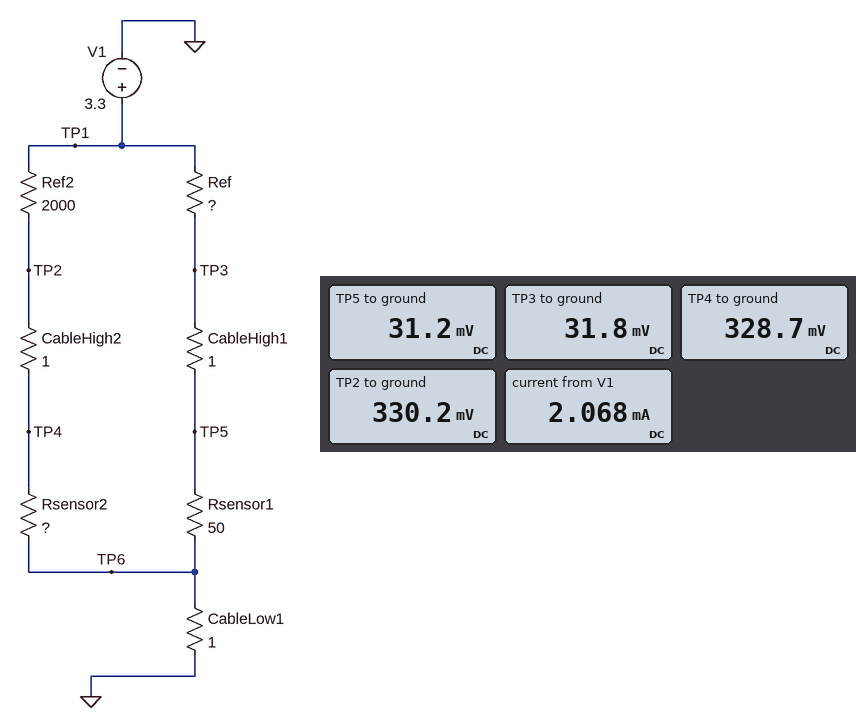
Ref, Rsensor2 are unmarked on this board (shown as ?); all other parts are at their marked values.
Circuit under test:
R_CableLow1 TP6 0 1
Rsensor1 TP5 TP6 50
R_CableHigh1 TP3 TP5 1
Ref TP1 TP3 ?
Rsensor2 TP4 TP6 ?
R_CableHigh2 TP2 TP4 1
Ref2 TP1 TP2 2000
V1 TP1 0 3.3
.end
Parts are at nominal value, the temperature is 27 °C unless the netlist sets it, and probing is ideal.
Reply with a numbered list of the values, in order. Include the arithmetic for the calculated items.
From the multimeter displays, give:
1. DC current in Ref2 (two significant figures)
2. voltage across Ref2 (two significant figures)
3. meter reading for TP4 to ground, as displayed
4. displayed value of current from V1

1. (3.3 V - 330.2 mV) / 2 kΩ = 1.5 mA
2. 3.3 V - 330.2 mV = 3.0 V
3. 328.7 mV
4. 2.068 mA
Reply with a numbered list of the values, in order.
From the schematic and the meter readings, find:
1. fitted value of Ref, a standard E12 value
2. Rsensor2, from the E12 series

1. 5.6 kΩ
2. 220 Ω
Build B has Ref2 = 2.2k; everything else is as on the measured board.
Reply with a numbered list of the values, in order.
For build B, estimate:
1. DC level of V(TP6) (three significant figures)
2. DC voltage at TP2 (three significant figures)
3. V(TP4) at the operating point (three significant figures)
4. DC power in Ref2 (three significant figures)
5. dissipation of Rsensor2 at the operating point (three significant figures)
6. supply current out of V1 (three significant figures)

1. 1.95 mV
2. 303 mV
3. 302 mV
4. 4.08 mW
5. 408 µW
6. 1.95 mA
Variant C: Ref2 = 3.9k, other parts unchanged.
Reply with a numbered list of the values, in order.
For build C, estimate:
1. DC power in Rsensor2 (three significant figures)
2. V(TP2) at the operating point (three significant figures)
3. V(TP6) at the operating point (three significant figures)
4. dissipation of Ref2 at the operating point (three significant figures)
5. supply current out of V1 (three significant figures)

1. 141 µW
2. 178 mV
3. 1.38 mV
4. 2.50 mW
5. 1.38 mA
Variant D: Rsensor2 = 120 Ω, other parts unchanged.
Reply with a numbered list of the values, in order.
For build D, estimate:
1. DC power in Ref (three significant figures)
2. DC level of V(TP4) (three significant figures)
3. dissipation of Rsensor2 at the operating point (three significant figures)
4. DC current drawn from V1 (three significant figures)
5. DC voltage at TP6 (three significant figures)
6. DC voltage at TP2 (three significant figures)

1. 1.91 mW
2. 189 mV
3. 290 µW
4. 2.14 mA
5. 2.14 mV
6. 190 mV
